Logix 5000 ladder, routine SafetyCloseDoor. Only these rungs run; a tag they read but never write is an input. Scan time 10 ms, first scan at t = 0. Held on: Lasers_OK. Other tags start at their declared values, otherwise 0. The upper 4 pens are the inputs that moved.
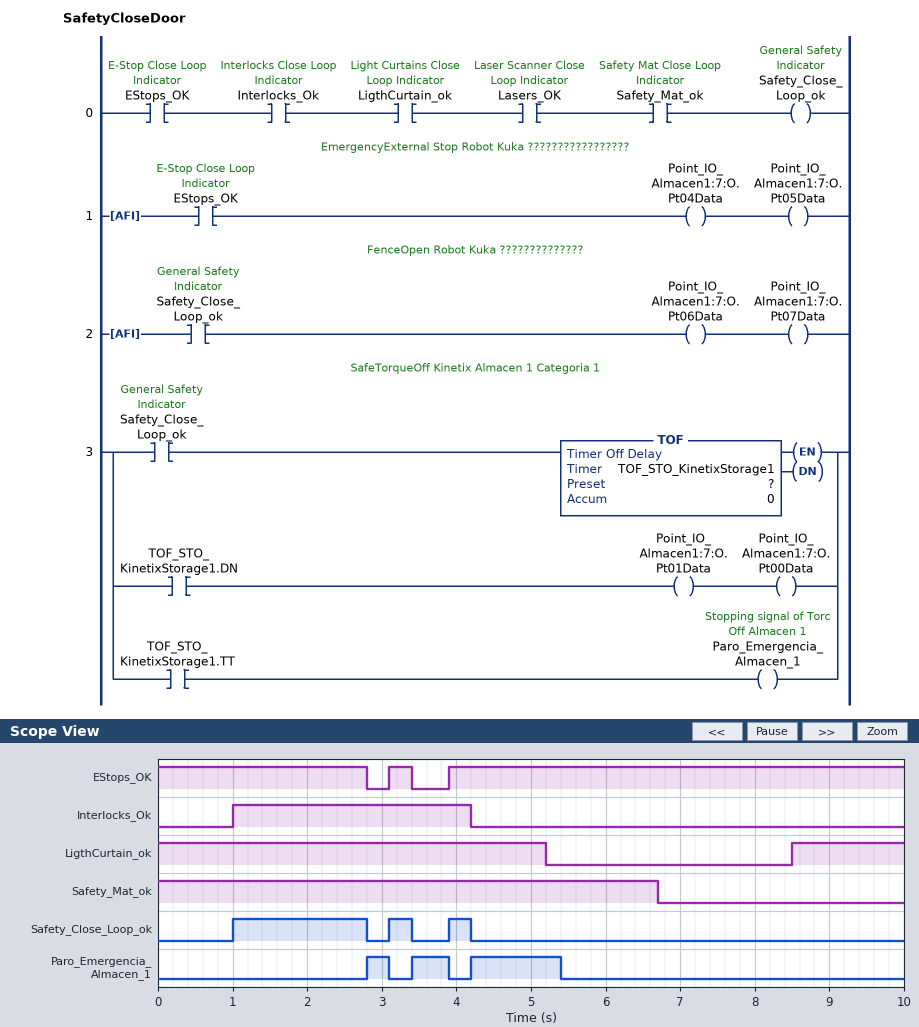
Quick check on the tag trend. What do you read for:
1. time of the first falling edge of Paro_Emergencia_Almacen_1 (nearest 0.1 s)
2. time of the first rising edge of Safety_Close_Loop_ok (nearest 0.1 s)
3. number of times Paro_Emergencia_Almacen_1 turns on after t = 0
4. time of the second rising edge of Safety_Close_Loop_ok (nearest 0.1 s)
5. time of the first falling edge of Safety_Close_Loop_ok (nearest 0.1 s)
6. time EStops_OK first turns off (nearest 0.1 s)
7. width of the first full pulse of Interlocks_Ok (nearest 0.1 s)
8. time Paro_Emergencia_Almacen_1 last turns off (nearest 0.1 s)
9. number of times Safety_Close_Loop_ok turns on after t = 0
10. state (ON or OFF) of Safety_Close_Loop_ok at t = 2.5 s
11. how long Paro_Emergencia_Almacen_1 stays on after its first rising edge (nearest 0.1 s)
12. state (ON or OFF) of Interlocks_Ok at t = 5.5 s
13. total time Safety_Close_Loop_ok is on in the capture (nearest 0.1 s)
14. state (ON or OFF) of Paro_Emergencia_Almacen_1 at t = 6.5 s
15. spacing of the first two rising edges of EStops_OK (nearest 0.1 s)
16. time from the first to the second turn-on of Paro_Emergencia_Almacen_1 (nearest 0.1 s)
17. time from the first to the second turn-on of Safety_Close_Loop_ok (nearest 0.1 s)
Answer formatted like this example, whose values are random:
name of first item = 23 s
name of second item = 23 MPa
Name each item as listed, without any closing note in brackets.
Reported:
time of the first falling edge of Paro_Emergencia_Almacen_1 = 3.1 s
time of the first rising edge of Safety_Close_Loop_ok = 1.0 s
number of times Paro_Emergencia_Almacen_1 turns on after t = 0 = 3
time of the second rising edge of Safety_Close_Loop_ok = 3.1 s
time of the first falling edge of Safety_Close_Loop_ok = 2.8 s
time EStops_OK first turns off = 2.8 s
width of the first full pulse of Interlocks_Ok = 3.2 s
time Paro_Emergencia_Almacen_1 last turns off = 5.4 s
number of times Safety_Close_Loop_ok turns on after t = 0 = 3
state (ON or OFF) of Safety_Close_Loop_ok at t = 2.5 s = ON
how long Paro_Emergencia_Almacen_1 stays on after its first rising edge = 0.3 s
state (ON or OFF) of Interlocks_Ok at t = 5.5 s = OFF
total time Safety_Close_Loop_ok is on in the capture = 2.4 s
state (ON or OFF) of Paro_Emergencia_Almacen_1 at t = 6.5 s = OFF
spacing of the first two rising edges of EStops_OK = 0.8 s
time from the first to the second turn-on of Paro_Emergencia_Almacen_1 = 0.6 s
time from the first to the second turn-on of Safety_Close_Loop_ok = 2.1 s
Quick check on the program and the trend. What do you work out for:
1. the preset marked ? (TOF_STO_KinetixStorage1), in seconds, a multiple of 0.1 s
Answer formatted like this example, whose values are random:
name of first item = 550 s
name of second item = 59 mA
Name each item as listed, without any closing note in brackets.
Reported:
the preset marked ? (TOF_STO_KinetixStorage1), in seconds, a multiple of 0.1 s = 1.2 s
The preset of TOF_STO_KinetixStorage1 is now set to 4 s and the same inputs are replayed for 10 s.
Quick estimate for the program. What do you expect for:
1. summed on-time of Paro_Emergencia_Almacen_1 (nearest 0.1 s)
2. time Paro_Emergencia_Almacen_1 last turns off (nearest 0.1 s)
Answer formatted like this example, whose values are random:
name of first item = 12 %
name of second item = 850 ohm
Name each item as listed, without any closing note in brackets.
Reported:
summed on-time of Paro_Emergencia_Almacen_1 = 4.8 s
time Paro_Emergencia_Almacen_1 last turns off = 8.2 s
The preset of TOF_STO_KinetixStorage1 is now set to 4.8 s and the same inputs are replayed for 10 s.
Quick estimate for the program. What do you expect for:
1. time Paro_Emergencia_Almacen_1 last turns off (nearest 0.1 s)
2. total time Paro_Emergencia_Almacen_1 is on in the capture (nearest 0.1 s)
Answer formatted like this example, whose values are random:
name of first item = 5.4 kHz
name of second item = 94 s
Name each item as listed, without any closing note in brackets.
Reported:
time Paro_Emergencia_Almacen_1 last turns off = 9.0 s
total time Paro_Emergencia_Almacen_1 is on in the capture = 5.6 s
